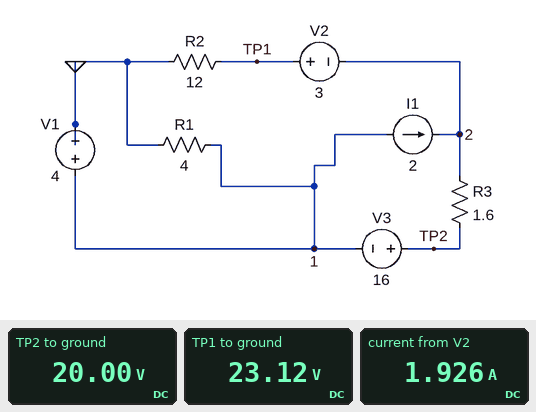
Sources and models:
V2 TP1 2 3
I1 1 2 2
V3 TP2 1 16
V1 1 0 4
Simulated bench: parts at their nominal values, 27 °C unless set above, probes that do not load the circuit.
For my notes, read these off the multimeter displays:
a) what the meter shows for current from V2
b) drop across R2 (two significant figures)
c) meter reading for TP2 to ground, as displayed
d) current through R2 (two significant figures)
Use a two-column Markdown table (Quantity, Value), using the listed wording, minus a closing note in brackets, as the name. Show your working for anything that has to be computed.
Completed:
| Quantity | Value |
|---|---|
| what the meter shows for current from V2 | 1.926 A |
| drop across R2 | 23.12 V = 23 V |
| meter reading for TP2 to ground, as displayed | 20.00 V |
| current through R2 | (23.12 V) / 12 Ω = 1.9 A |
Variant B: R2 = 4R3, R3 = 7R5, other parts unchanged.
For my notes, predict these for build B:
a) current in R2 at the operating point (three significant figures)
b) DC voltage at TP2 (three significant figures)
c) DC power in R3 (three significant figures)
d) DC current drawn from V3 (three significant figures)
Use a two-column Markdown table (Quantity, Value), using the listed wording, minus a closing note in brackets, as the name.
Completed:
| Quantity | Value |
|---|---|
| current in R2 at the operating point | 3.22 A |
| DC voltage at TP2 | 20.0 V |
| DC power in R3 | 11.2 W |
| DC current drawn from V3 | 1.22 A |
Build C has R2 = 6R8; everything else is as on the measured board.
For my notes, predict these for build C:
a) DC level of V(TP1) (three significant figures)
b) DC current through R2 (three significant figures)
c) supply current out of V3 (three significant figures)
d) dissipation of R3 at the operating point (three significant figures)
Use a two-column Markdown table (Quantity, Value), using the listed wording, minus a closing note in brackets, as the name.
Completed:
| Quantity | Value |
|---|---|
| DC level of V(TP1) | 21.2 V |
| DC current through R2 | 3.12 A |
| supply current out of V3 | 1.12 A |
| dissipation of R3 at the operating point | 2.00 W |
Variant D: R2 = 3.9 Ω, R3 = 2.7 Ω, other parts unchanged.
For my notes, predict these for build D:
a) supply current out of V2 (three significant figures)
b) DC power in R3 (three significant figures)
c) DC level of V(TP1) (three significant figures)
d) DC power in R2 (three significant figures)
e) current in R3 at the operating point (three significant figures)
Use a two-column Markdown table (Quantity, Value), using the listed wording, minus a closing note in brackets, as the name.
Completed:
| Quantity | Value |
|---|---|
| supply current out of V2 | 4.30 A |
| DC power in R3 | 14.3 W |
| DC level of V(TP1) | 16.8 V |
| DC power in R2 | 72.2 W |
| current in R3 at the operating point | 2.30 A |
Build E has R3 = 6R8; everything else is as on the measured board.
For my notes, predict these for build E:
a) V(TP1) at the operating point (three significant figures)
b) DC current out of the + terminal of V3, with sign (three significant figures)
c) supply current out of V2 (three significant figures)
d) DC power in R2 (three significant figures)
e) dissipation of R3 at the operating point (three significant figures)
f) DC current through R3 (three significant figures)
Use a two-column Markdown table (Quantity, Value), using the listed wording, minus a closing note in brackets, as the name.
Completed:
| Quantity | Value |
|---|---|
| V(TP1) at the operating point | 23.4 V |
| DC current out of the + terminal of V3, with sign | -53.2 mA |
| supply current out of V2 | 1.95 A |
| DC power in R2 | 45.5 W |
| dissipation of R3 at the operating point | 19.2 mW |
| DC current through R3 | 53.2 mA |
